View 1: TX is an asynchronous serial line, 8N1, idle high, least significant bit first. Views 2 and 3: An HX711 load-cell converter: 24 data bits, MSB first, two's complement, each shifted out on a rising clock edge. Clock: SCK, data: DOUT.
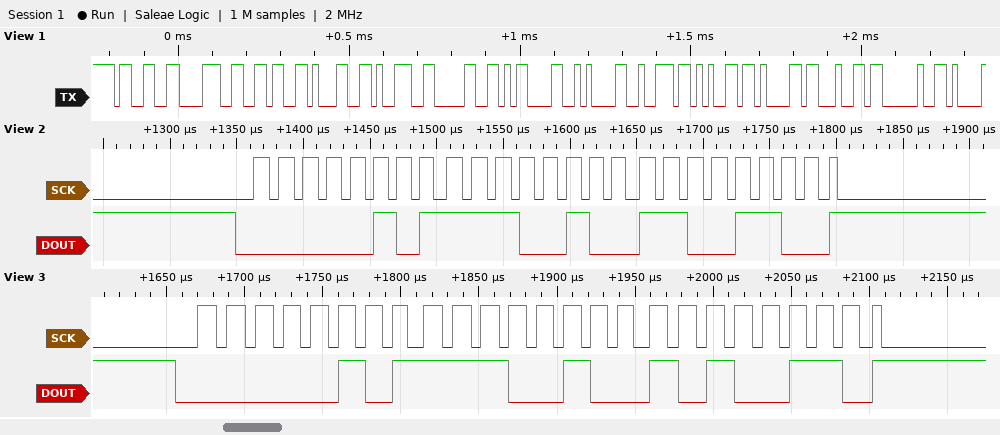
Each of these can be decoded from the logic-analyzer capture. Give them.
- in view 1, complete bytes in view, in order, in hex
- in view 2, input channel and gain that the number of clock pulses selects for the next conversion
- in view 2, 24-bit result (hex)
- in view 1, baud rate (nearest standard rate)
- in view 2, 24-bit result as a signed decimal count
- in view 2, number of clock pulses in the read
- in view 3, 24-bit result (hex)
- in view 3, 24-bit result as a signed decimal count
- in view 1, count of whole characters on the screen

33 38 36 31 39 30 0D 0A 72 65 61 64 20
channel A, gain 128
0x05E4CC
57600 baud
386252
25
0x05E4A6
386214
13
